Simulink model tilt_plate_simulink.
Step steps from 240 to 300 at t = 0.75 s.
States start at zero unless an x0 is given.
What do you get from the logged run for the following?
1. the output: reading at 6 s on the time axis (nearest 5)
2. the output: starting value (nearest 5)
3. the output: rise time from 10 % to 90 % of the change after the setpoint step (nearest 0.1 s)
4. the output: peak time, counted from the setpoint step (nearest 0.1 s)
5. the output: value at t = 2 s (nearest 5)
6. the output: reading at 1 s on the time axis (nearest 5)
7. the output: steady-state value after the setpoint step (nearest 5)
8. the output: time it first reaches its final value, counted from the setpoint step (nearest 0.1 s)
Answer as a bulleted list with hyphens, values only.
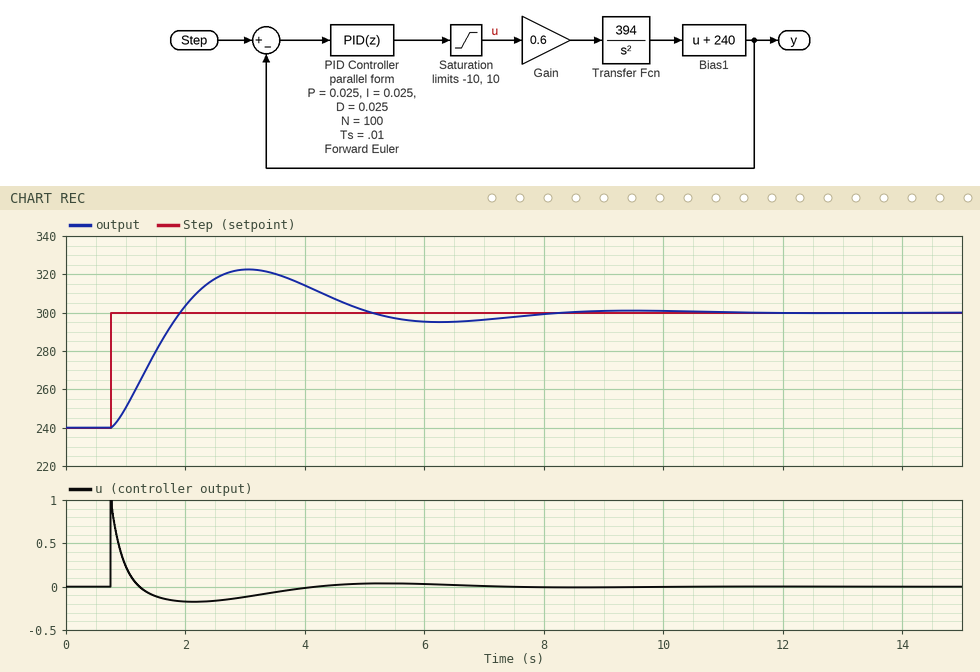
- 295
- 240
- 0.9 s
- 2.3 s
- 305
- 250
- 300
- 1.2 s
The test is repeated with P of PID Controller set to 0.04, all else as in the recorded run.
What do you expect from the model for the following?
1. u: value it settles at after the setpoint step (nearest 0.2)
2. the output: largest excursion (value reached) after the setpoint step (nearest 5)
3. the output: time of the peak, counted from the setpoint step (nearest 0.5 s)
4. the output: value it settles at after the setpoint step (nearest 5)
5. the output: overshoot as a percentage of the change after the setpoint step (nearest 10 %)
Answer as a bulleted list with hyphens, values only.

- 0.0
- 315
- 2.0 s
- 300
- 20 %
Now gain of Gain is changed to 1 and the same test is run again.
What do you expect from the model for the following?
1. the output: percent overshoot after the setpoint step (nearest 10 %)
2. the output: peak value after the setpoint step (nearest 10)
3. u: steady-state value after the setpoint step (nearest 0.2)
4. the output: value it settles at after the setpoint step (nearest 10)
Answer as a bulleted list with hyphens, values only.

- 30 %
- 320
- 0.0
- 300
